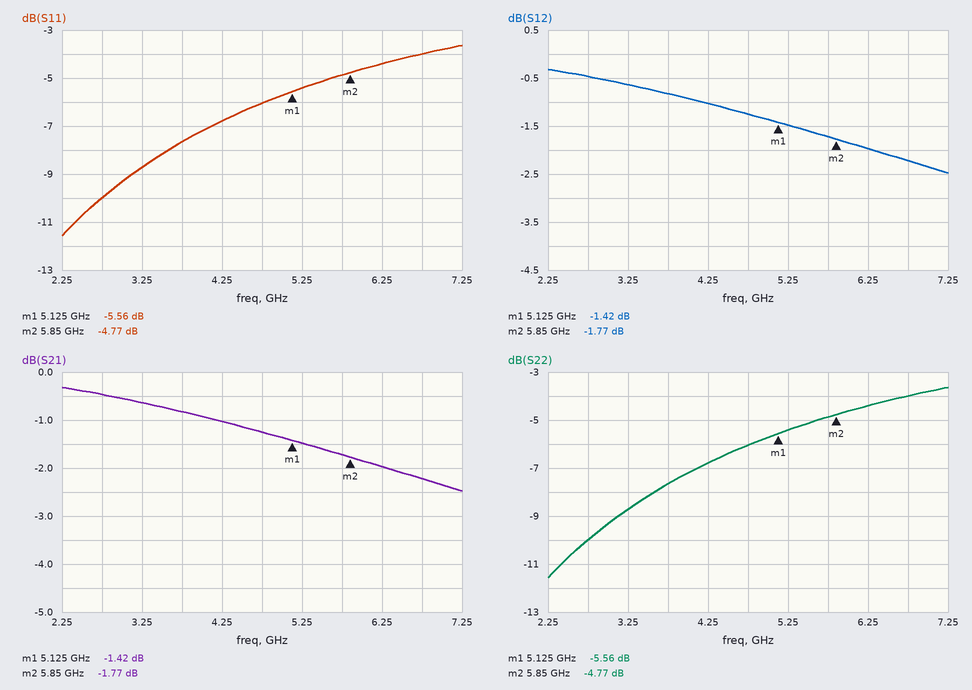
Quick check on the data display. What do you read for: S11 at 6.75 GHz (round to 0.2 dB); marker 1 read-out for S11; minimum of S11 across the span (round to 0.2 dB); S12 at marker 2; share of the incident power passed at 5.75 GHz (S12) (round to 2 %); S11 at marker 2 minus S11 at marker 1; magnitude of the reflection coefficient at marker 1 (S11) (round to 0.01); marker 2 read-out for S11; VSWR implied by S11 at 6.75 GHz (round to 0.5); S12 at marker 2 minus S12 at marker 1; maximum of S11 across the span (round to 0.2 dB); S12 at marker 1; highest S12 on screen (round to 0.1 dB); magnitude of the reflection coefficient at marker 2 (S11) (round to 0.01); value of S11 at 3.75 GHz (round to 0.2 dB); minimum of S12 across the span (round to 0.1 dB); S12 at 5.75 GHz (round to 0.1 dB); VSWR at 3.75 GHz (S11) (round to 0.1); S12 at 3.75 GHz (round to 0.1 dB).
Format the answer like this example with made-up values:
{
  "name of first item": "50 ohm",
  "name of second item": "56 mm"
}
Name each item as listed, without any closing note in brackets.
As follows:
{
  "S11 at 6.75 GHz": "-4.0 dB",
  "marker 1 read-out for S11": "-5.56 dB",
  "minimum of S11 across the span": "-11.6 dB",
  "S12 at marker 2": "-1.77 dB",
  "share of the incident power passed at 5.75 GHz (S12)": "68 %",
  "S11 at marker 2 minus S11 at marker 1": "0.79 dB",
  "magnitude of the reflection coefficient at marker 1 (S11)": "0.53",
  "marker 2 read-out for S11": "-4.77 dB",
  "VSWR implied by S11 at 6.75 GHz": "4.5",
  "S12 at marker 2 minus S12 at marker 1": "-0.35 dB",
  "maximum of S11 across the span": "-3.6 dB",
  "S12 at marker 1": "-1.42 dB",
  "highest S12 on screen": "-0.3 dB",
  "magnitude of the reflection coefficient at marker 2 (S11)": "0.58",
  "value of S11 at 3.75 GHz": "-7.6 dB",
  "minimum of S12 across the span": "-2.5 dB",
  "S12 at 5.75 GHz": "-1.7 dB",
  "VSWR at 3.75 GHz (S11)": "2.4",
  "S12 at 3.75 GHz": "-0.8 dB"
}
